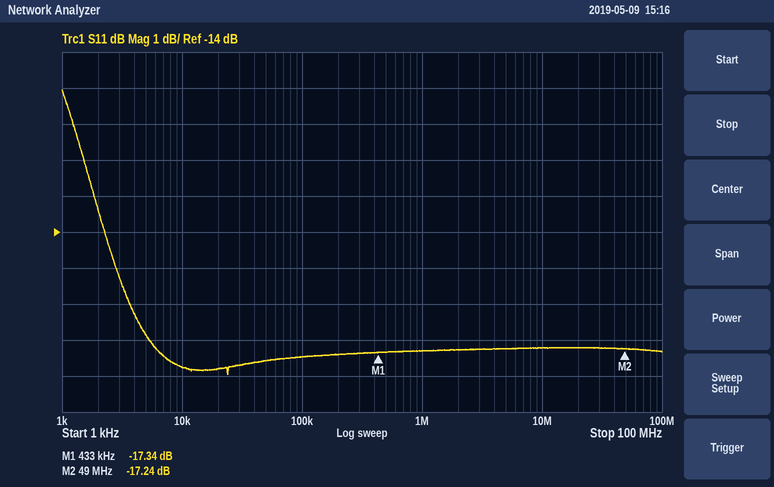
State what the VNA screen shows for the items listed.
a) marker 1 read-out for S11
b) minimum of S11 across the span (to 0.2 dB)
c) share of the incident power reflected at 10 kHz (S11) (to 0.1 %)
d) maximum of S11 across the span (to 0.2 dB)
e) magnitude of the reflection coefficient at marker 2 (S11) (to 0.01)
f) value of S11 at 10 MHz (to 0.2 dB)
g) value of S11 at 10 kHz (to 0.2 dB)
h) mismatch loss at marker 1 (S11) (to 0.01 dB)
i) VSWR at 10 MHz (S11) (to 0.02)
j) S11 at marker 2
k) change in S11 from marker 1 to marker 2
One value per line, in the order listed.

-17.34 dB
-18.0 dB
1.7 %
-10.0 dB
0.14
-17.2 dB
-17.8 dB
0.08 dB
1.32
-17.24 dB
0.10 dB
